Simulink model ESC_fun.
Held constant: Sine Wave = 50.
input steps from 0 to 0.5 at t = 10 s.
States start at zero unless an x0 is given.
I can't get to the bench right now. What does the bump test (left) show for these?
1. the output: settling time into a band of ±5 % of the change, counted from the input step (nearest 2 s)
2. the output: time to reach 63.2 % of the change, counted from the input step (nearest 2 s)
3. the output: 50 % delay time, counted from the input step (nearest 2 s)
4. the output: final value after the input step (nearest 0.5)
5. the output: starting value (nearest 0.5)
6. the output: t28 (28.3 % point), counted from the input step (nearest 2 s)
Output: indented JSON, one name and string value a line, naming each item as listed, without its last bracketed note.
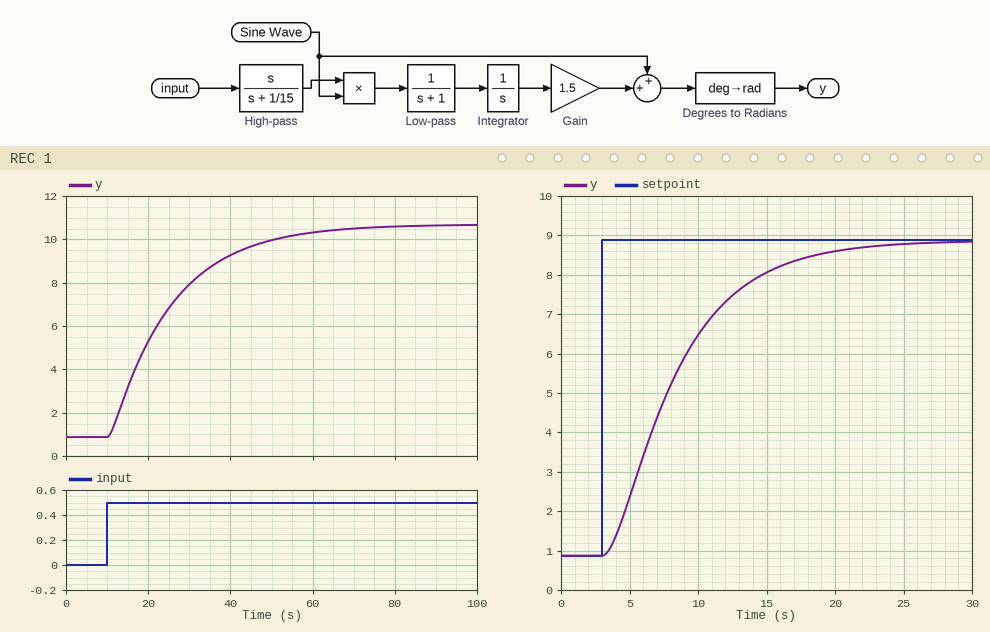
{
  "the output: settling time into a band of ±5 % of the change, counted from the input step": "46 s",
  "the output: time to reach 63.2 % of the change, counted from the input step": "16 s",
  "the output: 50 % delay time, counted from the input step": "12 s",
  "the output: final value after the input step": "10.5",
  "the output: starting value": "1.0",
  "the output: t28 (28.3 % point), counted from the input step": "6 s"
}
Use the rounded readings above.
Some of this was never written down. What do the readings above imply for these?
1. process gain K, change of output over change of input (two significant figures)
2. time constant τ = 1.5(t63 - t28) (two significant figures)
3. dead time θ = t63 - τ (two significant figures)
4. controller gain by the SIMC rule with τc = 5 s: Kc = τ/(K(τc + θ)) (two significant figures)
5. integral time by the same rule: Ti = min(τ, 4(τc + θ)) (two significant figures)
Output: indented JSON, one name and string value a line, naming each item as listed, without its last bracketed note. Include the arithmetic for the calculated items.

{
  "process gain K, change of output over change of input": "(10.5 - 1) / 0.5 = 19",
  "time constant τ = 1.5(t63 - t28)": "1.5 × (16 - 6) = 15 s",
  "dead time θ = t63 - τ": "16 - 15 = 1.0 s",
  "controller gain by the SIMC rule with τc = 5 s: Kc = τ/(K(τc + θ))": "15 / (19 × (5 + 1)) = 0.13",
  "integral time by the same rule: Ti = min(τ, 4(τc + θ))": "min(15, 4 × (5 + 1)) = 15 s"
}
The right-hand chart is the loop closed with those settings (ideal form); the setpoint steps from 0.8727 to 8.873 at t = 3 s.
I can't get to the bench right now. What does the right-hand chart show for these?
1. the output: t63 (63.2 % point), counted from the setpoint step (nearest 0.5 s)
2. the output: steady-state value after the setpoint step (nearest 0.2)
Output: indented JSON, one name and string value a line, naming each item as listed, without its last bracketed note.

{
  "the output: t63 (63.2 % point), counted from the setpoint step": "6.0 s",
  "the output: steady-state value after the setpoint step": "8.8"
}
